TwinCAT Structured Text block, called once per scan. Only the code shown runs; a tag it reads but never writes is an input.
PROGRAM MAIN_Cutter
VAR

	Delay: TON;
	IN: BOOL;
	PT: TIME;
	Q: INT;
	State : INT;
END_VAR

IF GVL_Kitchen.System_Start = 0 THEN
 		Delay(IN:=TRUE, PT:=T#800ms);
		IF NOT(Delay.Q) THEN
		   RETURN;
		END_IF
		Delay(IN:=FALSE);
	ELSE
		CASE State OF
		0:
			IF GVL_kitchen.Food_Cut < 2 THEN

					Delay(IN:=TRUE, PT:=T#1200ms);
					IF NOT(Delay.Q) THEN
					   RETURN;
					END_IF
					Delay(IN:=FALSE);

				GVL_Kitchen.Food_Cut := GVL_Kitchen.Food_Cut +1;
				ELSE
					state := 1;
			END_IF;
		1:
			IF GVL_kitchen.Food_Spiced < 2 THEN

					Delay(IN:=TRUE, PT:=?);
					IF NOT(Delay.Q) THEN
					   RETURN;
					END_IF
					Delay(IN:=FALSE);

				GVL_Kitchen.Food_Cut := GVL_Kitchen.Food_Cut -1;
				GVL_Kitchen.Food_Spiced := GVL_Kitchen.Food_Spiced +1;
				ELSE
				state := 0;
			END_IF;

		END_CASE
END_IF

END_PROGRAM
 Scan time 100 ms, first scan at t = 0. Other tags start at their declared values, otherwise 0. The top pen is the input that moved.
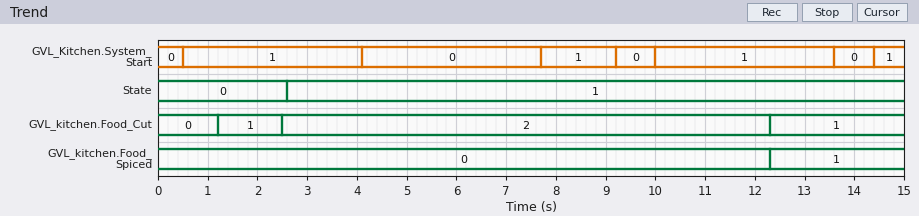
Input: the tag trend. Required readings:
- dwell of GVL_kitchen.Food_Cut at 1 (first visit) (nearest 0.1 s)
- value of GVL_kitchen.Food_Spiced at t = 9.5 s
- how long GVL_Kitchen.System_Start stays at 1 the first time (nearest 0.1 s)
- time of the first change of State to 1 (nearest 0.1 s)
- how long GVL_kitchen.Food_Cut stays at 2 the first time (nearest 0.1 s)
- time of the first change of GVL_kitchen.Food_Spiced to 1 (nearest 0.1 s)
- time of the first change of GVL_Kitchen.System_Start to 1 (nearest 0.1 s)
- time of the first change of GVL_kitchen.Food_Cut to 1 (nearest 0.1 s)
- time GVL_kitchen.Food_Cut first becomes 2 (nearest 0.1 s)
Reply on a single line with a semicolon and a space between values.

1.3 s; 0; 3.6 s; 2.6 s; 9.8 s; 12.3 s; 0.5 s; 1.2 s; 2.5 s
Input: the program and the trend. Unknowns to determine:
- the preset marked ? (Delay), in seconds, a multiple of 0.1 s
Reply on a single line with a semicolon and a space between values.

3.0 s
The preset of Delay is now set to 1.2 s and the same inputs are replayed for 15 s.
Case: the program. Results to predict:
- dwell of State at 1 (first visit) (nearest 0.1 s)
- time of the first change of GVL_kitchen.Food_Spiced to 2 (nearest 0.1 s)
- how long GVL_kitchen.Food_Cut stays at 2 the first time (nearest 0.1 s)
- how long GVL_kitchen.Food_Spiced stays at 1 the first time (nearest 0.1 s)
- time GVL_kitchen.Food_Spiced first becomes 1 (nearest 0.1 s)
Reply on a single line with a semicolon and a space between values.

6.3 s; 8.8 s; 1.4 s; 4.9 s; 3.9 s
